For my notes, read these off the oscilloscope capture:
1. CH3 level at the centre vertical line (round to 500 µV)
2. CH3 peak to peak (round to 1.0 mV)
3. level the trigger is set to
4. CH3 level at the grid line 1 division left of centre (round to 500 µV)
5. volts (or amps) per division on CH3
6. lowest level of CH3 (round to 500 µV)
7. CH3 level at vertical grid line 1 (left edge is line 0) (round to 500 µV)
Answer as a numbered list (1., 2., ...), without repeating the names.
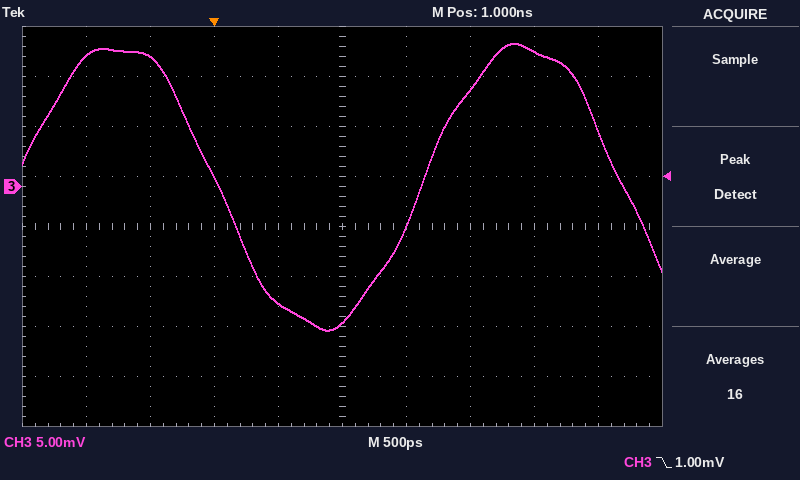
1. -13.5 mV
2. 29.0 mV
3. 1.00 mV
4. -11.5 mV
5. 5 mV
6. -14.5 mV
7. 13.0 mV
